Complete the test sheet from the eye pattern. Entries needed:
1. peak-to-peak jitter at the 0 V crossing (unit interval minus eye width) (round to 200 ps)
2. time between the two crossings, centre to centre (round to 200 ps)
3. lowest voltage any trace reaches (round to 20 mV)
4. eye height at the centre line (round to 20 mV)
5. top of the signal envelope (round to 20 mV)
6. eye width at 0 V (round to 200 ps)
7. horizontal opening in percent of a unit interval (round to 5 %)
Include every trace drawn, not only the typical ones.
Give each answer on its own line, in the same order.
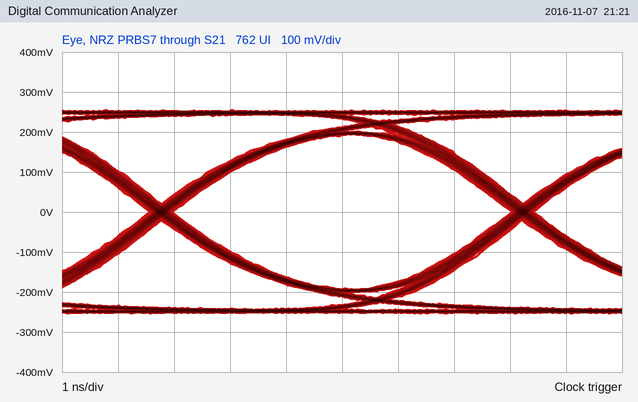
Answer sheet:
400 ps
6.4 ns
-260 mV
380 mV
260 mV
6.0 ns
95 %
